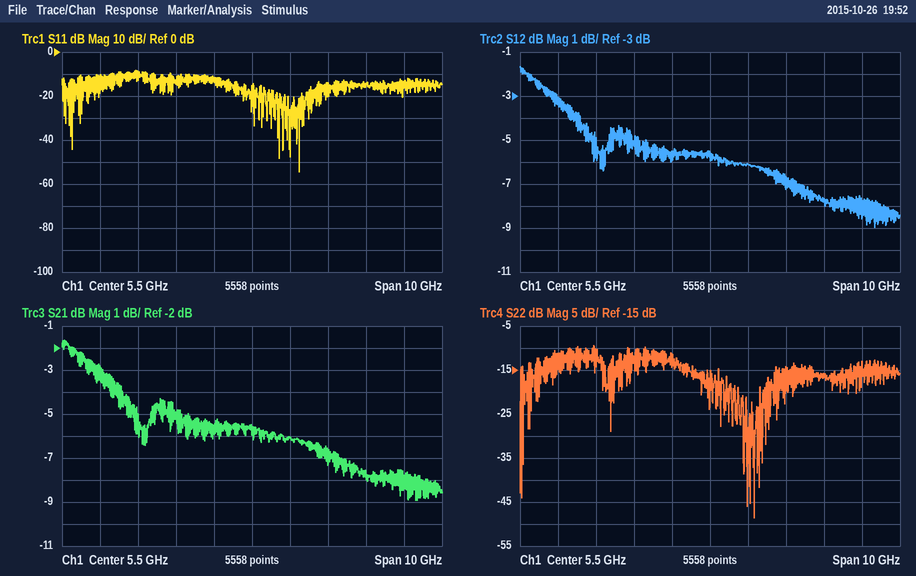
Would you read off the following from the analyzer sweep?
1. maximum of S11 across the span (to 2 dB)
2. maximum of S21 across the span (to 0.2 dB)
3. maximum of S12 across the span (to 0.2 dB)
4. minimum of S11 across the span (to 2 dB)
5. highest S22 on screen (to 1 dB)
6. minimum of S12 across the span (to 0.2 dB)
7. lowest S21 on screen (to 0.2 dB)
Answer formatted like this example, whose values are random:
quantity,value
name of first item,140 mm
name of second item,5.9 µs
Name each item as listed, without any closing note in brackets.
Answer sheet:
quantity,value
maximum of S11 across the span,-8 dB
maximum of S21 across the span,-1.6 dB
maximum of S12 across the span,-1.6 dB
minimum of S11 across the span,-54 dB
highest S22 on screen,-9 dB
minimum of S12 across the span,-9.0 dB
lowest S21 on screen,-9.0 dB
